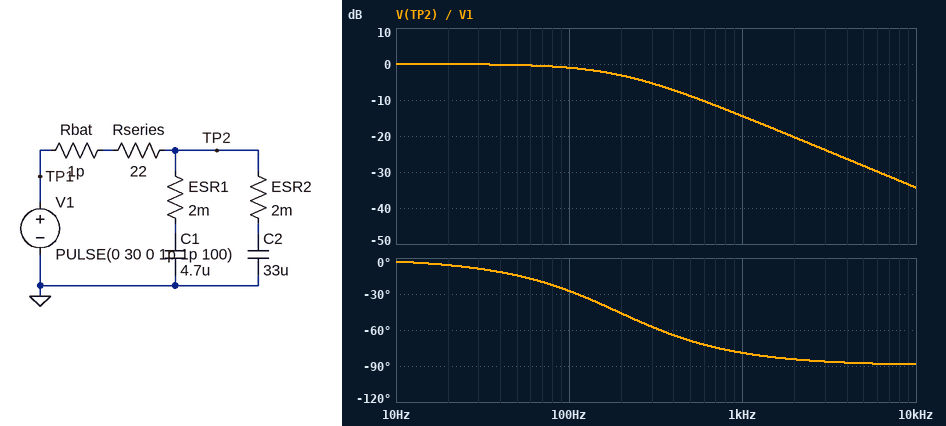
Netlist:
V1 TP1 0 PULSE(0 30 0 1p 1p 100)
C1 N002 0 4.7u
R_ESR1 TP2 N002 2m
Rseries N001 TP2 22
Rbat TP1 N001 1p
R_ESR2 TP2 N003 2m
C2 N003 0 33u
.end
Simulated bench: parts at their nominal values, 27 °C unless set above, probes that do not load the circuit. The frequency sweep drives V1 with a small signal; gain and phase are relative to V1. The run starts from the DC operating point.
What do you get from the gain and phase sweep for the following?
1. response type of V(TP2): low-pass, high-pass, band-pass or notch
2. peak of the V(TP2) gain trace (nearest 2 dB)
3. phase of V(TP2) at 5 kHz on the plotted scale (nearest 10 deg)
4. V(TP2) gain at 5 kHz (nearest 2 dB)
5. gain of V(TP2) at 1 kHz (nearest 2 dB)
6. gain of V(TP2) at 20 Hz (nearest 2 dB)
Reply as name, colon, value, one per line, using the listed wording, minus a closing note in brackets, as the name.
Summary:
response type of V(TP2): low-pass, high-pass, band-pass or notch: low-pass
peak of the V(TP2) gain trace: 0 dB
phase of V(TP2) at 5 kHz on the plotted scale: -90 deg
V(TP2) gain at 5 kHz: -28 dB
gain of V(TP2) at 1 kHz: -14 dB
gain of V(TP2) at 20 Hz: 0 dB
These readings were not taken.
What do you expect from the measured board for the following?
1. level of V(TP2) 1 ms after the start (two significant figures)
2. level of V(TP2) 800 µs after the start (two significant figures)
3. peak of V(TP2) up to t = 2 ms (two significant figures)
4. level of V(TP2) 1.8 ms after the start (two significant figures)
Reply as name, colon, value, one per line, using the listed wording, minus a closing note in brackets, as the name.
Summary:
level of V(TP2) 1 ms after the start: 21 V
level of V(TP2) 800 µs after the start: 19 V
peak of V(TP2) up to t = 2 ms: 27 V
level of V(TP2) 1.8 ms after the start: 27 V
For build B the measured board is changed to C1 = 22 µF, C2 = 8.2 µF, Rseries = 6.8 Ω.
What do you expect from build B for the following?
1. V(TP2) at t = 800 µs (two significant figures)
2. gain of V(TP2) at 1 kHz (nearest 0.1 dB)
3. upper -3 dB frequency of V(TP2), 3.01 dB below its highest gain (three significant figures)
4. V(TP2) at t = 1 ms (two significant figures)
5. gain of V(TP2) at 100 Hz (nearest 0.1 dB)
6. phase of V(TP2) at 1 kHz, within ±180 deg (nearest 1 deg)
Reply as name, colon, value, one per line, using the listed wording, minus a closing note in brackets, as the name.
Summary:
V(TP2) at t = 800 µs: 29 V
gain of V(TP2) at 1 kHz: -4.3 dB
upper -3 dB frequency of V(TP2), 3.01 dB below its highest gain: 775 Hz
V(TP2) at t = 1 ms: 30 V
gain of V(TP2) at 100 Hz: -0.1 dB
phase of V(TP2) at 1 kHz, within ±180 deg: -52 deg
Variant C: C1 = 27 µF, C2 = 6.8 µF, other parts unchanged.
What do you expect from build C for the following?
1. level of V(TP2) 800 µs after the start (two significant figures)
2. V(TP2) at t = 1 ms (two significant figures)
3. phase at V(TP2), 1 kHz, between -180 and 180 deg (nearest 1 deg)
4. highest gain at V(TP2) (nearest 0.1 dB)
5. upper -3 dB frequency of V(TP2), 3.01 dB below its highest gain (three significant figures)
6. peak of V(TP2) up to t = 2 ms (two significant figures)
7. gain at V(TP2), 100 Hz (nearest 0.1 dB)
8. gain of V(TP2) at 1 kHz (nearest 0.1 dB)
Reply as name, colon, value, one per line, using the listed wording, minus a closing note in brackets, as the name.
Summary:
level of V(TP2) 800 µs after the start: 20 V
V(TP2) at t = 1 ms: 22 V
phase at V(TP2), 1 kHz, between -180 and 180 deg: -78 deg
highest gain at V(TP2): 0 dB
upper -3 dB frequency of V(TP2), 3.01 dB below its highest gain: 214 Hz
peak of V(TP2) up to t = 2 ms: 28 V
gain at V(TP2), 100 Hz: -0.9 dB
gain of V(TP2) at 1 kHz: -13.6 dB
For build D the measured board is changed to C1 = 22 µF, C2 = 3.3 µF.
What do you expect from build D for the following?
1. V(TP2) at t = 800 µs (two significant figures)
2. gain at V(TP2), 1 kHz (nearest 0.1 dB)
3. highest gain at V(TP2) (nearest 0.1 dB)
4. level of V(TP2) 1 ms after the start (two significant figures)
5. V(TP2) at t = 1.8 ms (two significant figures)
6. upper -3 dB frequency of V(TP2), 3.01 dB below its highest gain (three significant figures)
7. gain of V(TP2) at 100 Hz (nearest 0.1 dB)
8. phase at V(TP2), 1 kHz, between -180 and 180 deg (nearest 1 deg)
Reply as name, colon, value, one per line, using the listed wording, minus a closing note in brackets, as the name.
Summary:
V(TP2) at t = 800 µs: 23 V
gain at V(TP2), 1 kHz: -11.2 dB
highest gain at V(TP2): 0 dB
level of V(TP2) 1 ms after the start: 25 V
V(TP2) at t = 1.8 ms: 29 V
upper -3 dB frequency of V(TP2), 3.01 dB below its highest gain: 286 Hz
gain of V(TP2) at 100 Hz: -0.5 dB
phase at V(TP2), 1 kHz, between -180 and 180 deg: -74 deg
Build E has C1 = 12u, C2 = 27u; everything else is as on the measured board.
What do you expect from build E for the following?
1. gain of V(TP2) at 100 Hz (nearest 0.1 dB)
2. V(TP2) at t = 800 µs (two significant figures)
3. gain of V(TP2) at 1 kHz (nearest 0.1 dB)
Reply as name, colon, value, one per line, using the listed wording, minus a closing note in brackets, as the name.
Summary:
gain of V(TP2) at 100 Hz: -1.1 dB
V(TP2) at t = 800 µs: 18 V
gain of V(TP2) at 1 kHz: -14.8 dB
